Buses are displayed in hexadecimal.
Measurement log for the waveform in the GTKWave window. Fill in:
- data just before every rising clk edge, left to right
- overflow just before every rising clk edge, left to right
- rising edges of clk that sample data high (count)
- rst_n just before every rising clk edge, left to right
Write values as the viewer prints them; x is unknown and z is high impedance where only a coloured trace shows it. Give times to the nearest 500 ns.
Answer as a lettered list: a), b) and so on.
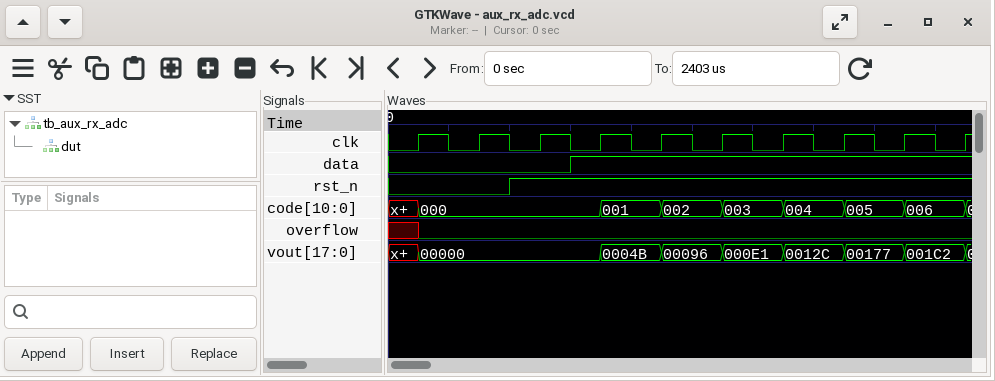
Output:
a) 0 0 0 1 1 1 1 1 1 1
b) x 0 0 0 0 0 0 0 0 0
c) 7
d) 0 0 1 1 1 1 1 1 1 1
